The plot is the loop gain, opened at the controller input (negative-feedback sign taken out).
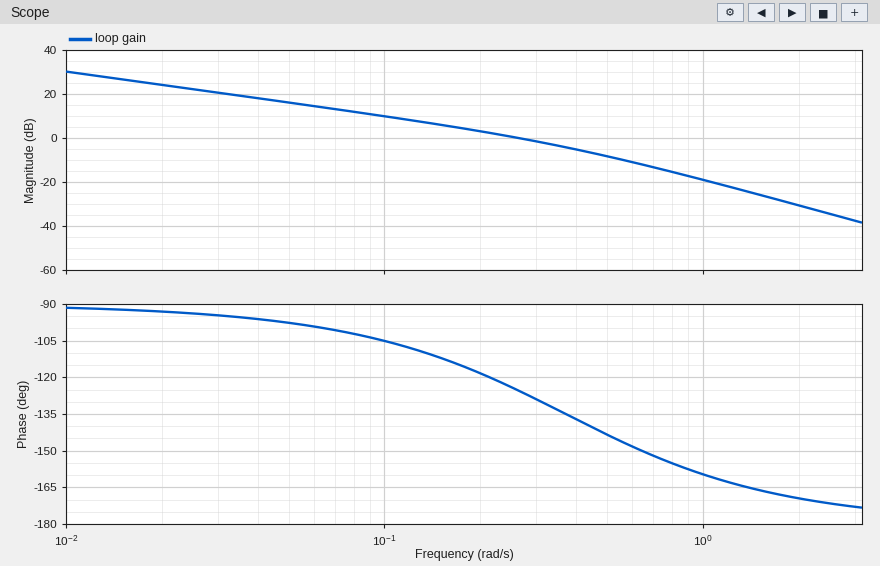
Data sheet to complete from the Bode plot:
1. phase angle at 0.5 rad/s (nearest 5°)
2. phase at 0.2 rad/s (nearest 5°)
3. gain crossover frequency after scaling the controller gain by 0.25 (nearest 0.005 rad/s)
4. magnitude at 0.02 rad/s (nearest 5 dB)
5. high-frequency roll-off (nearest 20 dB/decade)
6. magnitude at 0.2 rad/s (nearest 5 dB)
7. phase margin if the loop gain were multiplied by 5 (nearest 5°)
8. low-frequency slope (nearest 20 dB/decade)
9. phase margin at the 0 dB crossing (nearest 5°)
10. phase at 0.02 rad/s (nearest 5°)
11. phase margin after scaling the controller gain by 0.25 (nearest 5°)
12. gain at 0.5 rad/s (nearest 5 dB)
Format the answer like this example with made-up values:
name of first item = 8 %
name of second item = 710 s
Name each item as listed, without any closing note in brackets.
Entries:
phase angle at 0.5 rad/s = -145°
phase at 0.2 rad/s = -120°
gain crossover frequency after scaling the controller gain by 0.25 = 0.080 rad/s
magnitude at 0.02 rad/s = 25 dB
high-frequency roll-off = -40 dB/decade
magnitude at 0.2 rad/s = 5 dB
phase margin if the loop gain were multiplied by 5 = 25°
low-frequency slope = -20 dB/decade
phase margin at the 0 dB crossing = 55°
phase at 0.02 rad/s = -95°
phase margin after scaling the controller gain by 0.25 = 80°
gain at 0.5 rad/s = -10 dB
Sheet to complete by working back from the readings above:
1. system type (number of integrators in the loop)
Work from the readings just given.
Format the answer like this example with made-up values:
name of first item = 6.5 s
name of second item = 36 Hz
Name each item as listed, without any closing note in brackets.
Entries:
system type = 1
